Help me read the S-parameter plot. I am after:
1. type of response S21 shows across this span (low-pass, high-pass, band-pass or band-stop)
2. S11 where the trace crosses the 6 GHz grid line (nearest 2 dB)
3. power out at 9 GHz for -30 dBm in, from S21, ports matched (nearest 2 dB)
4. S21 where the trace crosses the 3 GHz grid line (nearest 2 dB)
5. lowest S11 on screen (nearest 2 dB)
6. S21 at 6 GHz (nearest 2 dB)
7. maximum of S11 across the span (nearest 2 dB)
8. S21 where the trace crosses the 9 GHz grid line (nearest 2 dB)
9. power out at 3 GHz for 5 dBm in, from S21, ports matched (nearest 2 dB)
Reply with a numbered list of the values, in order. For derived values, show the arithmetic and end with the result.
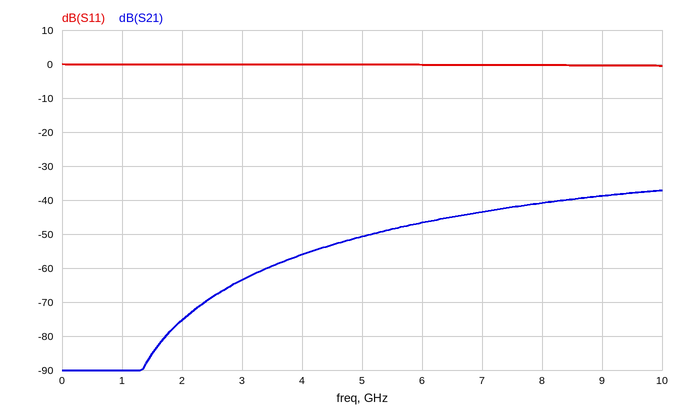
1. high-pass
2. 0 dB
3. -30 dBm + (-38 dB) = -68 dBm
4. -64 dB
5. 0 dB
6. -46 dB
7. 0 dB
8. -38 dB
9. 5 dBm + (-64 dB) = -58 dBm
